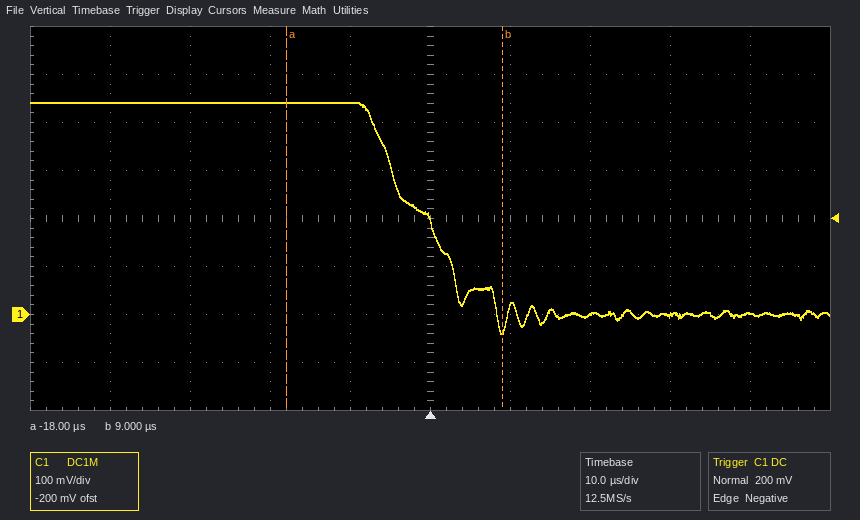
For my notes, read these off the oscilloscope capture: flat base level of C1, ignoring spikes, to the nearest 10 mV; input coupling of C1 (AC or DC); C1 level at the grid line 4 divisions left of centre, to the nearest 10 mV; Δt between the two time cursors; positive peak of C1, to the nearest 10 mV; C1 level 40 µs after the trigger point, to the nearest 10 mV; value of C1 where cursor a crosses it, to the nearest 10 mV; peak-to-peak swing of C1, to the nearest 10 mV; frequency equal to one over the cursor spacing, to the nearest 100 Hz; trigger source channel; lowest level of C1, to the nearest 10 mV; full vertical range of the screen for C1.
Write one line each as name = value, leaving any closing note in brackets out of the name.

flat base level of C1, ignoring spikes, to the nearest 10 mV = 0 mV
input coupling of C1 = DC
C1 level at the grid line 4 divisions left of centre, to the nearest 10 mV = 440 mV
Δt between the two time cursors = 27 µs
positive peak of C1, to the nearest 10 mV = 440 mV
C1 level 40 µs after the trigger point, to the nearest 10 mV = 0 mV
value of C1 where cursor a crosses it, to the nearest 10 mV = 440 mV
peak-to-peak swing of C1, to the nearest 10 mV = 480 mV
frequency equal to one over the cursor spacing, to the nearest 100 Hz = 37.0 kHz
trigger source channel = C1
lowest level of C1, to the nearest 10 mV = -40 mV
full vertical range of the screen for C1 = 800 mV
